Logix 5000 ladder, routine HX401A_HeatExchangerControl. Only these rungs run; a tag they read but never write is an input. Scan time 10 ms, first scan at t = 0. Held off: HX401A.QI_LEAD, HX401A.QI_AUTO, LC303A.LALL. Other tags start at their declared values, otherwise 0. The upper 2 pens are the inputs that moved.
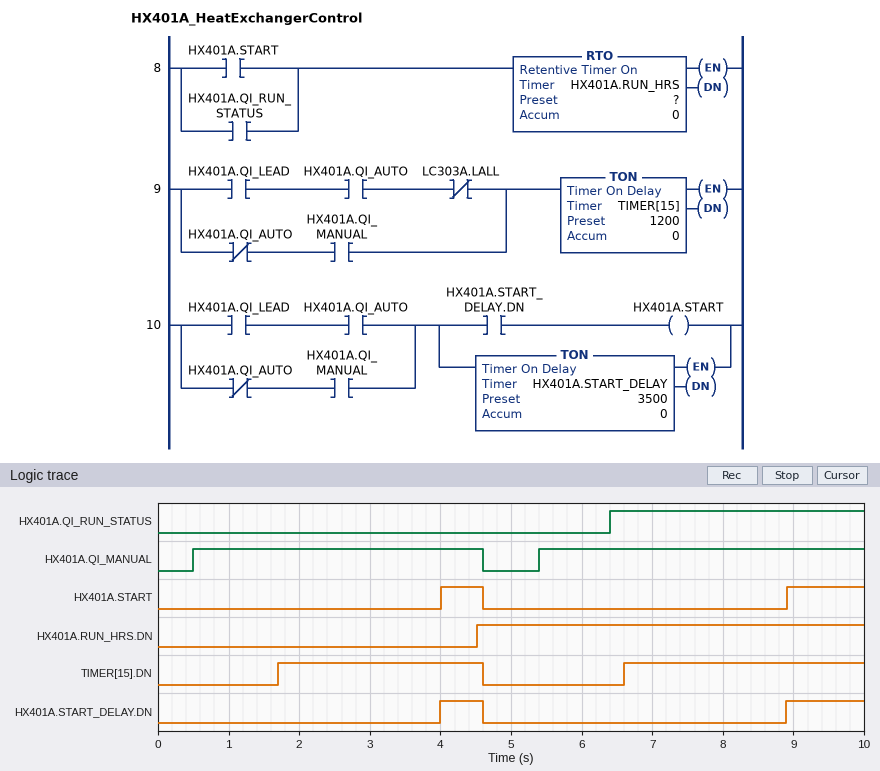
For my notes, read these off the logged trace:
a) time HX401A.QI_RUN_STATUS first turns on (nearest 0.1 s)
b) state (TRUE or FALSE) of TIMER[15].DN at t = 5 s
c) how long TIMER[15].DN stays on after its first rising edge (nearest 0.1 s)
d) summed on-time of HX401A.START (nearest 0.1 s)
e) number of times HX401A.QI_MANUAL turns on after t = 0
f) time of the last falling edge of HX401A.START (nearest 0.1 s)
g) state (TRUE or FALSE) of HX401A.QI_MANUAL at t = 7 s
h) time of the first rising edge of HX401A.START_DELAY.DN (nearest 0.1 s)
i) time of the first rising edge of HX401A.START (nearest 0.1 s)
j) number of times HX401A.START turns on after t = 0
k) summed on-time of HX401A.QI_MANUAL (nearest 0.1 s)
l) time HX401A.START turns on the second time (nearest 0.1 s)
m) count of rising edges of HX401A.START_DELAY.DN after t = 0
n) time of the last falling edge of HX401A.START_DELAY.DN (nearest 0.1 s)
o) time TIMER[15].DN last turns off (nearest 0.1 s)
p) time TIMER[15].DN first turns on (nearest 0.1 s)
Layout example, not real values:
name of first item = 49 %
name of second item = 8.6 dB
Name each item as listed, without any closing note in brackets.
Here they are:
time HX401A.QI_RUN_STATUS first turns on = 6.4 s
state (TRUE or FALSE) of TIMER[15].DN at t = 5 s = FALSE
how long TIMER[15].DN stays on after its first rising edge = 2.9 s
summed on-time of HX401A.START = 1.7 s
number of times HX401A.QI_MANUAL turns on after t = 0 = 2
time of the last falling edge of HX401A.START = 4.6 s
state (TRUE or FALSE) of HX401A.QI_MANUAL at t = 7 s = TRUE
time of the first rising edge of HX401A.START_DELAY.DN = 4.0 s
time of the first rising edge of HX401A.START = 4.0 s
number of times HX401A.START turns on after t = 0 = 2
summed on-time of HX401A.QI_MANUAL = 8.7 s
time HX401A.START turns on the second time = 8.9 s
count of rising edges of HX401A.START_DELAY.DN after t = 0 = 2
time of the last falling edge of HX401A.START_DELAY.DN = 4.6 s
time TIMER[15].DN last turns off = 4.6 s
time TIMER[15].DN first turns on = 1.7 s
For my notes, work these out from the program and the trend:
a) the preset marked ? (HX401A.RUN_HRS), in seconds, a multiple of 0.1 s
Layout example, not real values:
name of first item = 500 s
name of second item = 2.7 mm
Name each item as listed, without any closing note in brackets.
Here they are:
the preset marked ? (HX401A.RUN_HRS), in seconds, a multiple of 0.1 s = 0.5 s
